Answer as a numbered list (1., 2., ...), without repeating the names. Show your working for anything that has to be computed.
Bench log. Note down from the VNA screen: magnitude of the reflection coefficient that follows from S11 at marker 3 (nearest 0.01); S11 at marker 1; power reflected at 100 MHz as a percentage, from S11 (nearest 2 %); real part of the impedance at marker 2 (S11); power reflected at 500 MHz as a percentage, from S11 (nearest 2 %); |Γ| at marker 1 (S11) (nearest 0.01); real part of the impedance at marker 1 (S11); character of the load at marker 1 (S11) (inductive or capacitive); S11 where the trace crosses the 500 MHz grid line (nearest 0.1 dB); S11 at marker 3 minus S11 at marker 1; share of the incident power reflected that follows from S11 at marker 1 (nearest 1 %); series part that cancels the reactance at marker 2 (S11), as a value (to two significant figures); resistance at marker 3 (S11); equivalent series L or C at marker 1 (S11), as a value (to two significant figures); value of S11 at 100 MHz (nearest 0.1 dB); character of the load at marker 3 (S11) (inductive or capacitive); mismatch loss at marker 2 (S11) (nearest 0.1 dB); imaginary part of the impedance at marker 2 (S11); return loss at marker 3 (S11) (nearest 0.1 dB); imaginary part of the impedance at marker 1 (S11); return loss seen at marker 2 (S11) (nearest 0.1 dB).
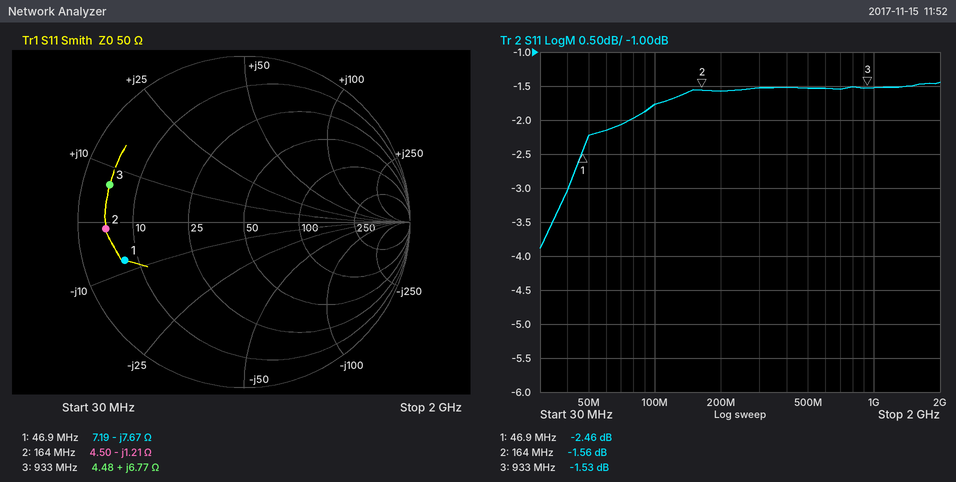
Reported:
1. 10^(-1.53/20) ≈ 0.84
2. -2.46 dB
3. 10^(-1.8/10) ≈ 66 %
4. 4.50 Ω
5. 10^(-1.5/10) ≈ 70.8 %, so 70 % to the nearest 2 %
6. 0.75
7. 7.19 Ω
8. capacitive
9. -1.5 dB
10. -1.53 − (-2.46) = 0.93 dB
11. 10^(-2.46/10) ≈ 57 %
12. L = 1.21 Ω/(2π × 164 MHz) ≈ 1.2 nH
13. 4.48 Ω
14. C = 1/(2π × 46.9 MHz × 7.67 Ω) ≈ 442 pF, so 440 pF to two significant figures
15. -1.8 dB
16. inductive
17. −10 log10(1 − 10^(-1.56/10)) ≈ 5.2 dB
18. -1.21 Ω
19. 1.5 dB
20. -7.67 Ω
21. 1.6 dB
